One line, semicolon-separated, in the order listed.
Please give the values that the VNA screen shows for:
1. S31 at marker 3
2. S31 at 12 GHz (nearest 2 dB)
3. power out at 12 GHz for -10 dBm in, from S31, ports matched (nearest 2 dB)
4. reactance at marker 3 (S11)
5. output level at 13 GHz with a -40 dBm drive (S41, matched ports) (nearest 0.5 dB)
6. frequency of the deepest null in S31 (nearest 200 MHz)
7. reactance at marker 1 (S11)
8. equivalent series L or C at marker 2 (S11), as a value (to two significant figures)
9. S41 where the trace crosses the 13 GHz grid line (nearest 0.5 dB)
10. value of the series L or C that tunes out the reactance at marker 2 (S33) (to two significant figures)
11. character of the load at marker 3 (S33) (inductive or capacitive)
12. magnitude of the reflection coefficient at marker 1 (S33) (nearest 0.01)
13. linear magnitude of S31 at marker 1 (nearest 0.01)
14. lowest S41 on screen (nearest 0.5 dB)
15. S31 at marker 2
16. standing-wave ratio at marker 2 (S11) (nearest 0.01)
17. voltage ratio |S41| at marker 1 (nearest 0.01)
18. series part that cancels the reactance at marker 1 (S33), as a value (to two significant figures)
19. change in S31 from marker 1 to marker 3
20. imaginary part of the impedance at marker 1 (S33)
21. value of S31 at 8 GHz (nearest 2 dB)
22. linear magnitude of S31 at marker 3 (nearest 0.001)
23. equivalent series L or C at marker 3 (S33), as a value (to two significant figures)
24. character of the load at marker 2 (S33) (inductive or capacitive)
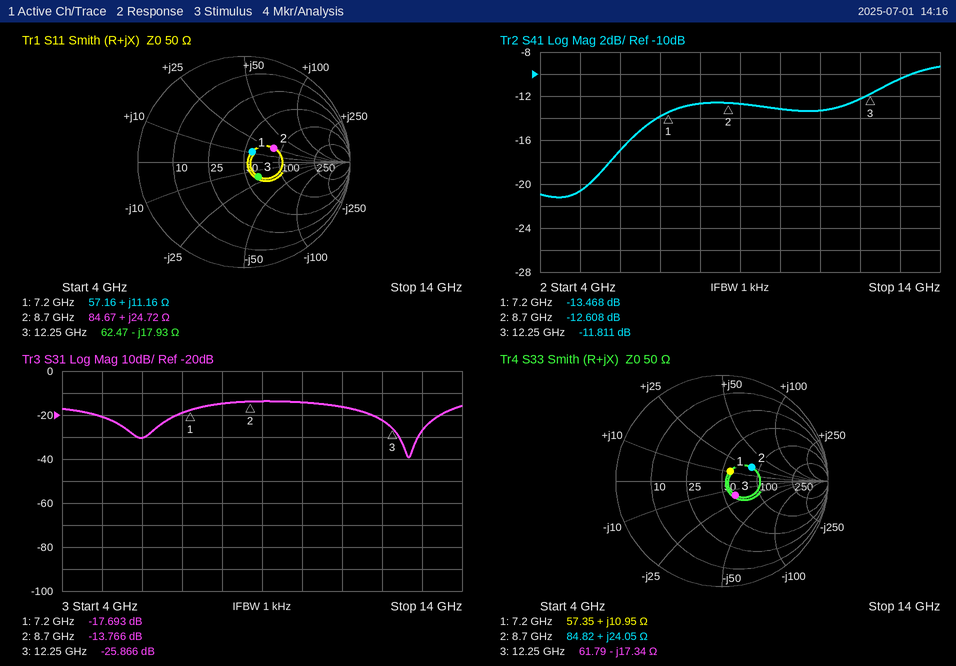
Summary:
-25.866 dB; -22 dB; -32 dBm; -17.93 Ω; -50.5 dBm; 12.6 GHz; +11.16 Ω; 450 pH; -10.5 dB; 760 fF; capacitive; 0.12; 0.13; -21.0 dB; -13.766 dB; 1.90; 0.21; 2.0 pF; -8.173 dB; +10.95 Ω; -14 dB; 0.051; 750 fF; inductive
